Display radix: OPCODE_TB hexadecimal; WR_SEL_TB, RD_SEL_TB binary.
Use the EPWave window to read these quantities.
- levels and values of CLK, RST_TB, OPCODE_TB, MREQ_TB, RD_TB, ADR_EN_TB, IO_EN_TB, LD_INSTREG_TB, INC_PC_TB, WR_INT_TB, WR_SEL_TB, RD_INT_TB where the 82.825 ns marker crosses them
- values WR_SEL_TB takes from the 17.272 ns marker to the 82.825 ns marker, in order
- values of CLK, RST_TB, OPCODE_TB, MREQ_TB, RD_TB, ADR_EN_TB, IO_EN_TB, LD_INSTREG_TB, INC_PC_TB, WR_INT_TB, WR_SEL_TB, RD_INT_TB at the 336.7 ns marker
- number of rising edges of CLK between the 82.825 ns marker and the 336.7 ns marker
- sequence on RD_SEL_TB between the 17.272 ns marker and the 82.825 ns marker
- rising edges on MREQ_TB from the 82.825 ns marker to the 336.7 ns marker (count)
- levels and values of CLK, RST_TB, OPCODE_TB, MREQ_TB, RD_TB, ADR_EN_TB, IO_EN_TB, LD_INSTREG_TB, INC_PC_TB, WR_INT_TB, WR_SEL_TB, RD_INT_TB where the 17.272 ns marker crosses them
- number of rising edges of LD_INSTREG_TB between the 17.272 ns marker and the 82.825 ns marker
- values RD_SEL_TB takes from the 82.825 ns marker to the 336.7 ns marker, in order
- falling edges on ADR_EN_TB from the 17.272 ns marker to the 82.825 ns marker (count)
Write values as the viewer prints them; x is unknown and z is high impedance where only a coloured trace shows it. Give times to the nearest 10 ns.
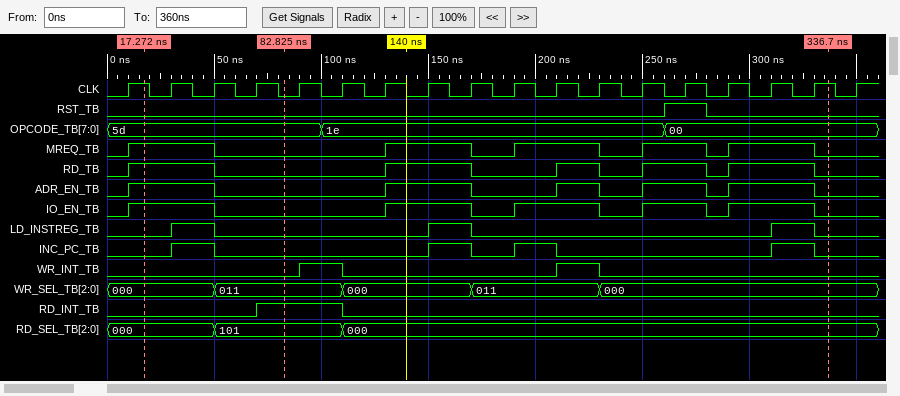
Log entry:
CLK=0, RST_TB=0, OPCODE_TB=5d, MREQ_TB=0, RD_TB=0, ADR_EN_TB=0, IO_EN_TB=0, LD_INSTREG_TB=0, INC_PC_TB=0, WR_INT_TB=0, WR_SEL_TB=011, RD_INT_TB=1
000, 011
CLK=1, RST_TB=0, OPCODE_TB=00, MREQ_TB=0, RD_TB=0, ADR_EN_TB=0, IO_EN_TB=0, LD_INSTREG_TB=0, INC_PC_TB=0, WR_INT_TB=0, WR_SEL_TB=000, RD_INT_TB=0
13
000, 101
4
CLK=1, RST_TB=0, OPCODE_TB=5d, MREQ_TB=1, RD_TB=1, ADR_EN_TB=1, IO_EN_TB=1, LD_INSTREG_TB=0, INC_PC_TB=0, WR_INT_TB=0, WR_SEL_TB=000, RD_INT_TB=0
1
101, 000
1
